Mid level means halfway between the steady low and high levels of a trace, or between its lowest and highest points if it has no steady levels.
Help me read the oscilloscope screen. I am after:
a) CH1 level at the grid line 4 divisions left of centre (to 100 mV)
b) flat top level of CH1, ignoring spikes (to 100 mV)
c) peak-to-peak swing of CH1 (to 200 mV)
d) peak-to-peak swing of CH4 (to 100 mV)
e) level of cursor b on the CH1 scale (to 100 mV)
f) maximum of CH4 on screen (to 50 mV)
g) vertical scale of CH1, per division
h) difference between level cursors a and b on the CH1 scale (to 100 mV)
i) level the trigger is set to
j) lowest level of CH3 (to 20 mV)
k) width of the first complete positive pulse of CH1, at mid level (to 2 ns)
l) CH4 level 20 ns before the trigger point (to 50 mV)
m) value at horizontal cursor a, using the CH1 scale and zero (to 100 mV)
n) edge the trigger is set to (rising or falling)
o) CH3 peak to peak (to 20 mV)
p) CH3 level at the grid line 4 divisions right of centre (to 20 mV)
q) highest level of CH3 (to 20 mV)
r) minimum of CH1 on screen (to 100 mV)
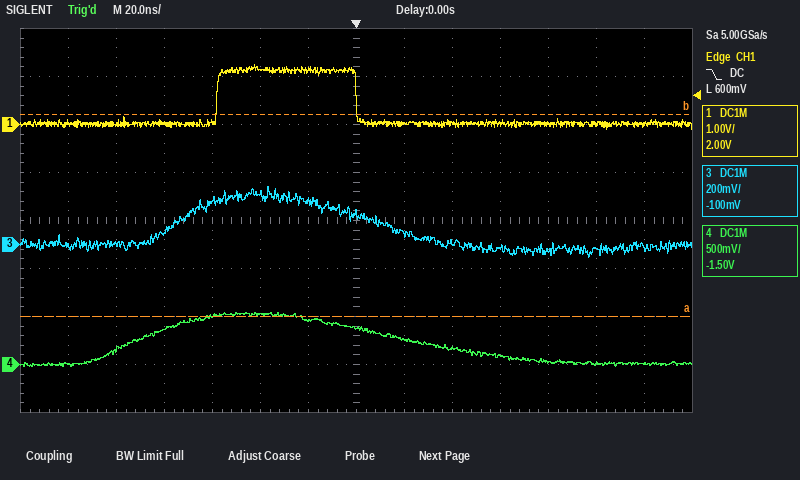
0.0 V
1.1 V
1.4 V
600 mV
200 mV
550 mV
1 V
4.2 V
600 mV
-60 mV
58 ns
450 mV
-4.0 V
falling
300 mV
-20 mV
240 mV
-100 mV
